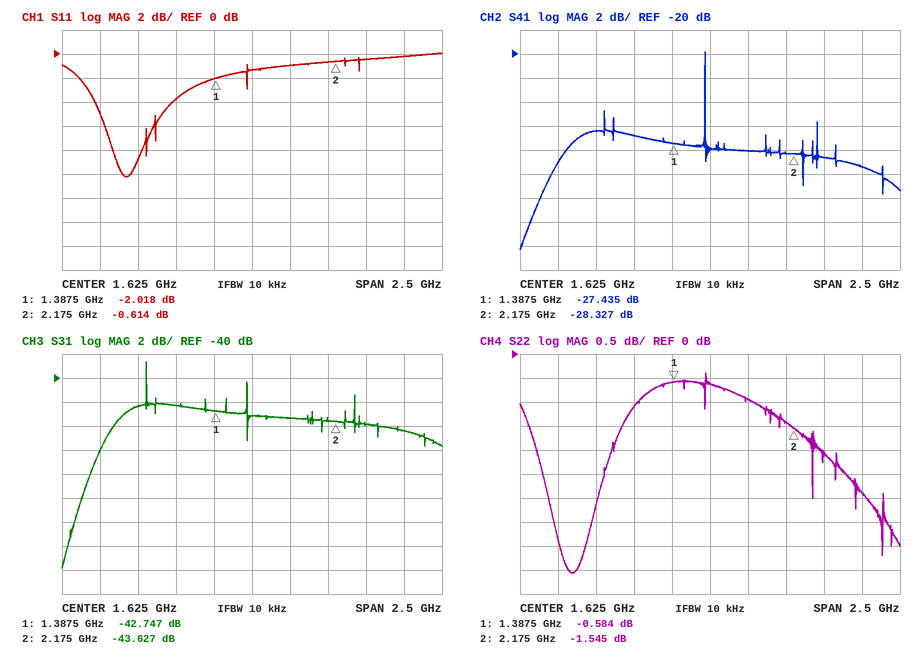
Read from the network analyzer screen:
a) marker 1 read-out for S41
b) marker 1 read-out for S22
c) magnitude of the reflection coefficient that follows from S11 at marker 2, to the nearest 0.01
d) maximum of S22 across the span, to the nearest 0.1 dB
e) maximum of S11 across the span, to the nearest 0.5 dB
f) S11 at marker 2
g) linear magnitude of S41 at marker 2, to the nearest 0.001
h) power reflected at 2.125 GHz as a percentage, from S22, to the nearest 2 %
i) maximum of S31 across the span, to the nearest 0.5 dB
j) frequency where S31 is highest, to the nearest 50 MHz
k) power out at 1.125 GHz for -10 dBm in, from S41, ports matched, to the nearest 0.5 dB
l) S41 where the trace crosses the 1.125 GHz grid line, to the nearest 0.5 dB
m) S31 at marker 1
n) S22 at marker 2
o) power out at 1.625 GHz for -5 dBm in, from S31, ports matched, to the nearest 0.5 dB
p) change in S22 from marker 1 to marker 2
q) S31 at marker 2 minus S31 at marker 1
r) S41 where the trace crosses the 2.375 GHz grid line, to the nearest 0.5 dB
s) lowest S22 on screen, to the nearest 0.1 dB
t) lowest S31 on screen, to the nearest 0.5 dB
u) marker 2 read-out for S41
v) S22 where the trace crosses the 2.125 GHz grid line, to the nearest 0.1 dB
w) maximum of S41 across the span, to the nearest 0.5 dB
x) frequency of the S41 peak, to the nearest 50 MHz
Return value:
-27.435 dB
-0.584 dB
0.93
-0.4 dB
0.0 dB
-0.614 dB
0.038
72 %
-38.5 dB
950 MHz
-37.0 dBm
-27.0 dB
-42.747 dB
-1.545 dB
-48.0 dBm
-0.961 dB
-0.880 dB
-28.5 dB
-4.6 dB
-56.0 dB
-28.327 dB
-1.4 dB
-20.0 dB
1.60 GHz
